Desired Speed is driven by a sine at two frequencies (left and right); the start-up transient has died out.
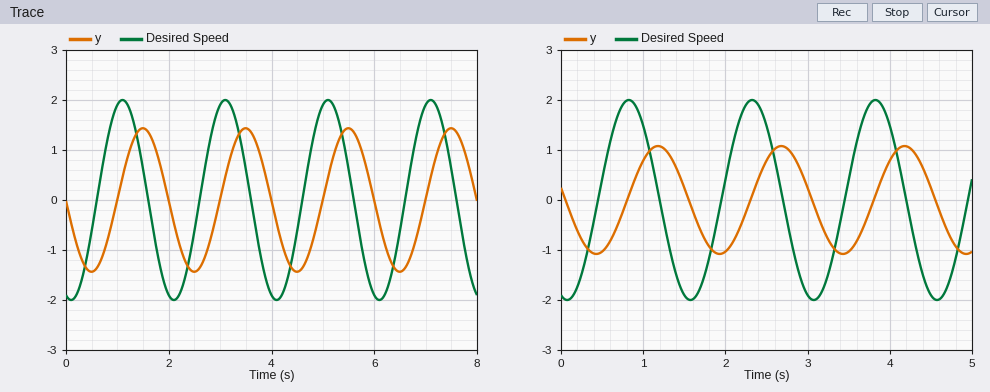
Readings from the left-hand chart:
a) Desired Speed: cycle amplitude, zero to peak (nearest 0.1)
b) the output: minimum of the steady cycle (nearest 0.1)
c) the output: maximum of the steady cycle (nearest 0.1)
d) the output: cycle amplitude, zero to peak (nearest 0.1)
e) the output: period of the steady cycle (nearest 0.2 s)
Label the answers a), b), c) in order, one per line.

a) 2.0
b) -1.4
c) 1.4
d) 1.4
e) 2.0 s
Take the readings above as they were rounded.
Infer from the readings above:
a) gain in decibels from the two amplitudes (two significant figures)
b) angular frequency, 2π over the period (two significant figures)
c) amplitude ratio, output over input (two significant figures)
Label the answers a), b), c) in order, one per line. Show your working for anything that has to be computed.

a) 20 log10(1.4 / 2) = -3.1 dB
b) 2π / 2 = 3.1 rad/s
c) 1.4 / 2 = 0.70
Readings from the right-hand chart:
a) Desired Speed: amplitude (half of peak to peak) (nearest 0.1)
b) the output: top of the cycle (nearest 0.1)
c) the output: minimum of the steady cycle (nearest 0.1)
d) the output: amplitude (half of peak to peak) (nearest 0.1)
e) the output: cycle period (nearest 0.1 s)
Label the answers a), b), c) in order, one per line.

a) 2.0
b) 1.1
c) -1.1
d) 1.1
e) 1.5 s
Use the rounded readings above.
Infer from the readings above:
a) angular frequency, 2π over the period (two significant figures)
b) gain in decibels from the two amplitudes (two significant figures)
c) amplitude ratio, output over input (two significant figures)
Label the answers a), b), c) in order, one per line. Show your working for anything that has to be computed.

a) 2π / 1.5 = 4.2 rad/s
b) 20 log10(1.1 / 2) = -5.2 dB
c) 1.1 / 2 = 0.55
